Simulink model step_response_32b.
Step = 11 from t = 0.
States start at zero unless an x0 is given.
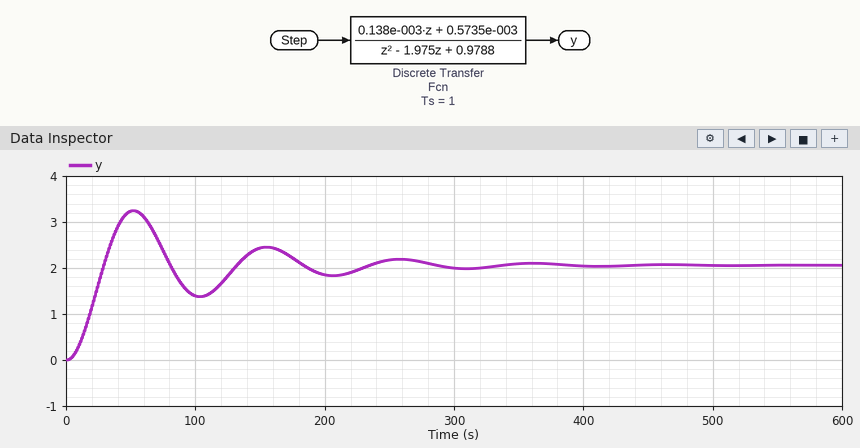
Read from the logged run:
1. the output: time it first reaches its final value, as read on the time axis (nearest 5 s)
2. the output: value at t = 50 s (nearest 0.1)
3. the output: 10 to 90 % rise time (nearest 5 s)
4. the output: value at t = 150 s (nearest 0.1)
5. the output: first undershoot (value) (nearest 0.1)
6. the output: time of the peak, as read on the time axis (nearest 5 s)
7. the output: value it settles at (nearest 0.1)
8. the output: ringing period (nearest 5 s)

30 s
3.2
20 s
2.4
1.4
50 s
2.1
105 s
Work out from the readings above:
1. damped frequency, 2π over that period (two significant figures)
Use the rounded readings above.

0.060 rad/s
